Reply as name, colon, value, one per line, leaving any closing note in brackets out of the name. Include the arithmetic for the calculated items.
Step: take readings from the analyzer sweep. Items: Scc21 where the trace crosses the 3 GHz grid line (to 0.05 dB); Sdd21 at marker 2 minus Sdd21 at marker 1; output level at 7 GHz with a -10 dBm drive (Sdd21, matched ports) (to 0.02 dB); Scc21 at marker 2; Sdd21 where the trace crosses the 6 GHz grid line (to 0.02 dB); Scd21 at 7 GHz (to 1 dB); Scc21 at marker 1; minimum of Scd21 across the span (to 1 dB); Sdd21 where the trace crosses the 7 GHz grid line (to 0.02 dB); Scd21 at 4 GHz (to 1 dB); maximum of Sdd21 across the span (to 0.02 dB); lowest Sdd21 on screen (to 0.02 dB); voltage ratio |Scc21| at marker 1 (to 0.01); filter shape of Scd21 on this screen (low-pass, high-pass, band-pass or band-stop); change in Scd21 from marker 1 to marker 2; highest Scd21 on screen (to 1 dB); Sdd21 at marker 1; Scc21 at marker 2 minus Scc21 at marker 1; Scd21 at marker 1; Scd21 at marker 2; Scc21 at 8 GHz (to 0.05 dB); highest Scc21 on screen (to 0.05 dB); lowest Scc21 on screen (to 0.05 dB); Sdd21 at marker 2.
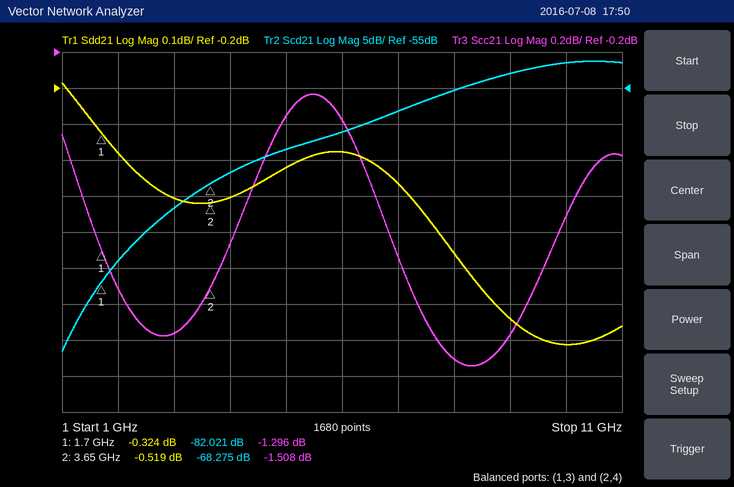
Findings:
Scc21 where the trace crosses the 3 GHz grid line: -1.75 dB
Sdd21 at marker 2 minus Sdd21 at marker 1: -0.519 − (-0.324) = -0.195 dB
output level at 7 GHz with a -10 dBm drive (Sdd21, matched ports): -10 dBm + (-0.46 dB) = -10.46 dBm
Scc21 at marker 2: -1.508 dB
Sdd21 where the trace crosses the 6 GHz grid line: -0.38 dB
Scd21 at 7 GHz: -58 dB
Scc21 at marker 1: -1.296 dB
minimum of Scd21 across the span: -92 dB
Sdd21 where the trace crosses the 7 GHz grid line: -0.46 dB
Scd21 at 4 GHz: -67 dB
maximum of Sdd21 across the span: -0.18 dB
lowest Sdd21 on screen: -0.92 dB
voltage ratio |Scc21| at marker 1: 10^(-1.296/20) ≈ 0.86
filter shape of Scd21 on this screen: high-pass
change in Scd21 from marker 1 to marker 2: -68.275 − (-82.021) = 13.746 dB
highest Scd21 on screen: -51 dB
Sdd21 at marker 1: -0.324 dB
Scc21 at marker 2 minus Scc21 at marker 1: -1.508 − (-1.296) = -0.212 dB
Scd21 at marker 1: -82.021 dB
Scd21 at marker 2: -68.275 dB
Scc21 at 8 GHz: -1.90 dB
highest Scc21 on screen: -0.45 dB
lowest Scc21 on screen: -1.95 dB
Sdd21 at marker 2: -0.519 dB
